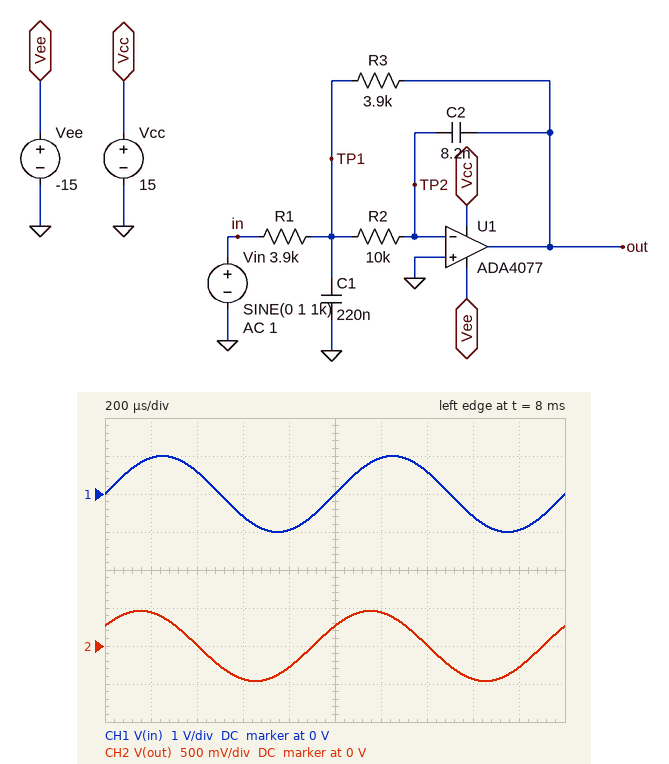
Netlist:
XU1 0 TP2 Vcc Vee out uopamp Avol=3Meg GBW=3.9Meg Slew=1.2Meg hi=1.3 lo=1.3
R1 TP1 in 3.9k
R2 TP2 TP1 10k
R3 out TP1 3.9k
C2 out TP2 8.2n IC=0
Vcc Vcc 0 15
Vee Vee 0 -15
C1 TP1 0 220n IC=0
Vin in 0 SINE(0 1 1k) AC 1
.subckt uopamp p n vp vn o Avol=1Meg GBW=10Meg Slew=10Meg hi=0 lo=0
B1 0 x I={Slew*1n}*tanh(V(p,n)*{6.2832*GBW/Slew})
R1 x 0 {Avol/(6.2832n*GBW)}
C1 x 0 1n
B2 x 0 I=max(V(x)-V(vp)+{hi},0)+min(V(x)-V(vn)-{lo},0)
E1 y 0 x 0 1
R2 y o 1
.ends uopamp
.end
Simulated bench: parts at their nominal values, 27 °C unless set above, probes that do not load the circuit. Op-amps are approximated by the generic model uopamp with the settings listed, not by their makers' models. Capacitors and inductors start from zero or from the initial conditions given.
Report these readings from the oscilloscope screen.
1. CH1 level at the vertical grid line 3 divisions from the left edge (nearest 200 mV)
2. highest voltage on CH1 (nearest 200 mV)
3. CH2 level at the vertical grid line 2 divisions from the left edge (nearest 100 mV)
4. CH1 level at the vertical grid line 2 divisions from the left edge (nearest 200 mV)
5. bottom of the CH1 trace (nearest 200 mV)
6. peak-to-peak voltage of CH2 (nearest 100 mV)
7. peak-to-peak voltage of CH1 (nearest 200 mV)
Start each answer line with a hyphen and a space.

- -600 mV
- 1.0 V
- 0 V
- 600 mV
- -1.0 V
- 900 mV
- 2.0 V
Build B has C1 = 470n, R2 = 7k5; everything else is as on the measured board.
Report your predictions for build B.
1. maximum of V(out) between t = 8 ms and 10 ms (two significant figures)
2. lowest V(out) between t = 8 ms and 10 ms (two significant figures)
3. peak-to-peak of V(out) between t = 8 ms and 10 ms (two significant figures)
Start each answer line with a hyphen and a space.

- 280 mV
- -280 mV
- 560 mV
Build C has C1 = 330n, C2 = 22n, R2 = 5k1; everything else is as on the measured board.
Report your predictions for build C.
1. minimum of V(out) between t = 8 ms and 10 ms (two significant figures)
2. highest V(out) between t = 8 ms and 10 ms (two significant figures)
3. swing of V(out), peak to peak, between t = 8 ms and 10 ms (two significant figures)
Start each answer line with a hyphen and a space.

- -200 mV
- 200 mV
- 390 mV
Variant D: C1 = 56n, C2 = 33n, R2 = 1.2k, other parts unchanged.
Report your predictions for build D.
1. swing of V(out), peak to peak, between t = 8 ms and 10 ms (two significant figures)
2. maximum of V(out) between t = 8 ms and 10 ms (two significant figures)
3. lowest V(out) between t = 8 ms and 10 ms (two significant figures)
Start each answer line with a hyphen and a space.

- 1.4 V
- 680 mV
- -680 mV
